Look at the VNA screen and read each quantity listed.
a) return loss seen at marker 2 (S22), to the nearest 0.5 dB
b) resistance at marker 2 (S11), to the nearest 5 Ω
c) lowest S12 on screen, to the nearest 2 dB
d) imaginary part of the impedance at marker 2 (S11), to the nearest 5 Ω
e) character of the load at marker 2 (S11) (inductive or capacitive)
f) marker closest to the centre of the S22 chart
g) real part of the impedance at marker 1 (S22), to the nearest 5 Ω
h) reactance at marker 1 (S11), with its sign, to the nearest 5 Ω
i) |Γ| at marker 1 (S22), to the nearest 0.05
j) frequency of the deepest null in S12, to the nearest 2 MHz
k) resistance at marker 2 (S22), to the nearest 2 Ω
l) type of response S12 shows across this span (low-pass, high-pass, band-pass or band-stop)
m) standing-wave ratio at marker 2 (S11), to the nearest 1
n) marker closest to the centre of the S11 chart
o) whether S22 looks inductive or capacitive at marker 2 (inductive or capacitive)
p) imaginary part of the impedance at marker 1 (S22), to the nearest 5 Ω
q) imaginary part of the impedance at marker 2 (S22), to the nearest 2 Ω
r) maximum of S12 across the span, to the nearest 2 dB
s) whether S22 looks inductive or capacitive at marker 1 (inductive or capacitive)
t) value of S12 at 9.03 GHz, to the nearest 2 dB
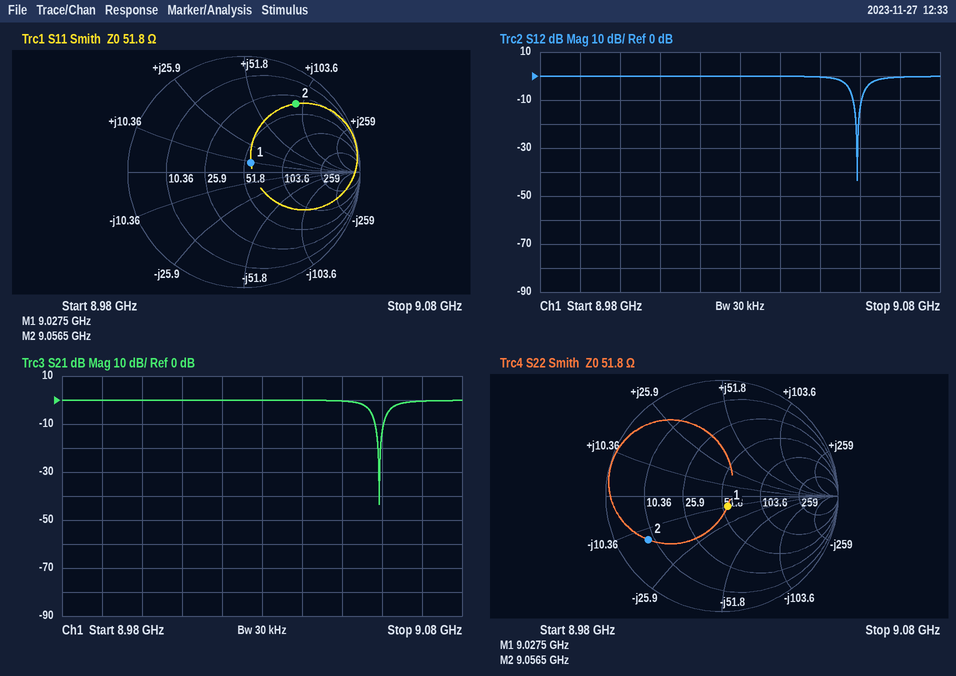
2.5 dB
35 Ω
-44 dB
+95 Ω
inductive
marker 1
55 Ω
+10 Ω
0.10
9.060 GHz
8 Ω
band-stop
7
marker 1
capacitive
-10 Ω
-14 Ω
0 dB
capacitive
0 dB
